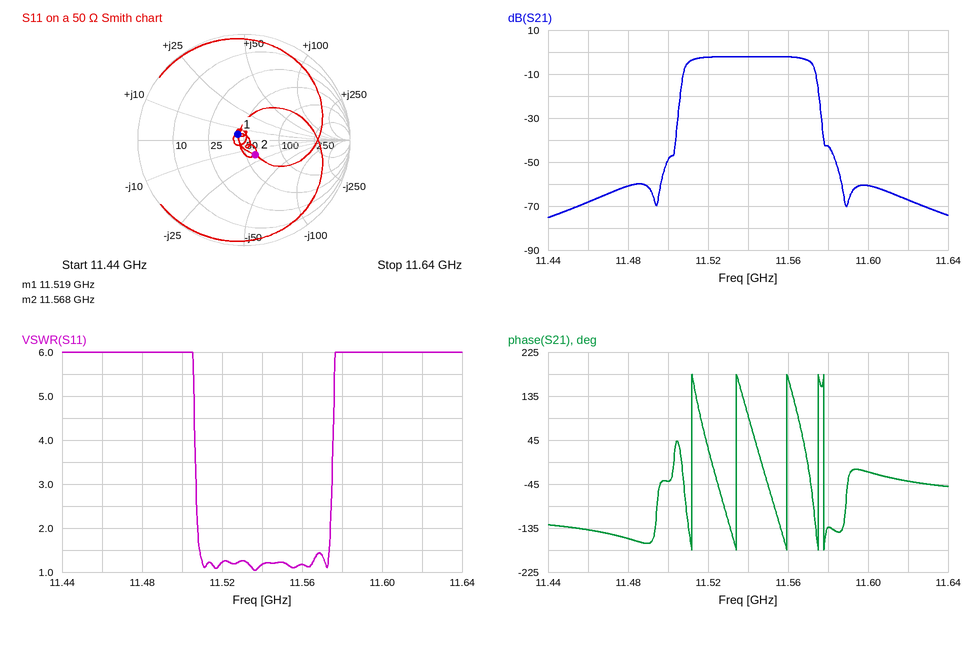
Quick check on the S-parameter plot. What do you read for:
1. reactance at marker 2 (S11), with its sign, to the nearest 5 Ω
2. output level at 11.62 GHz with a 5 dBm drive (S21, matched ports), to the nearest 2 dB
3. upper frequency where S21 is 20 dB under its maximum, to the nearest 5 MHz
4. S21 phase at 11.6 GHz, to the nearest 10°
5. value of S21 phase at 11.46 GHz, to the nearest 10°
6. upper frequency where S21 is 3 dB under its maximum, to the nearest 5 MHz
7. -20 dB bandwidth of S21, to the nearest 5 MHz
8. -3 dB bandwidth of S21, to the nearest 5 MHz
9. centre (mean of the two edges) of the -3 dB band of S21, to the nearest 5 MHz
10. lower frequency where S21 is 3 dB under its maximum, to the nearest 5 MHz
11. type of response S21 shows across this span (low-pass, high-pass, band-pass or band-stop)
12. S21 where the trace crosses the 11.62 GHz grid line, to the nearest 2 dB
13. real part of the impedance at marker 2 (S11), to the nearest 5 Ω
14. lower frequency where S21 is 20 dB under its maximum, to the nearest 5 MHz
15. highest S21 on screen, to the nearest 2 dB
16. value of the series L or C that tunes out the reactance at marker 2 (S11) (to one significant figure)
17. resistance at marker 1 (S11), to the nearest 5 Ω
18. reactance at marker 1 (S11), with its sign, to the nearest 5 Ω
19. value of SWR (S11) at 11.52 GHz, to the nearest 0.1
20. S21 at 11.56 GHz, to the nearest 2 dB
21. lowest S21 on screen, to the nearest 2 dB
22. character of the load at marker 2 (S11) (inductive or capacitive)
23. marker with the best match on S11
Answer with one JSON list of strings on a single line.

["-15 Ω", "-62 dBm", "11.575 GHz", "-20°", "-140°", "11.570 GHz", "70 MHz", "60 MHz", "11.540 GHz", "11.510 GHz", "band-pass", "-68 dB", "60 Ω", "11.505 GHz", "-2 dB", "200 pH", "45 Ω", "+5 Ω", "1.2", "-2 dB", "-76 dB", "capacitive", "marker 1"]
